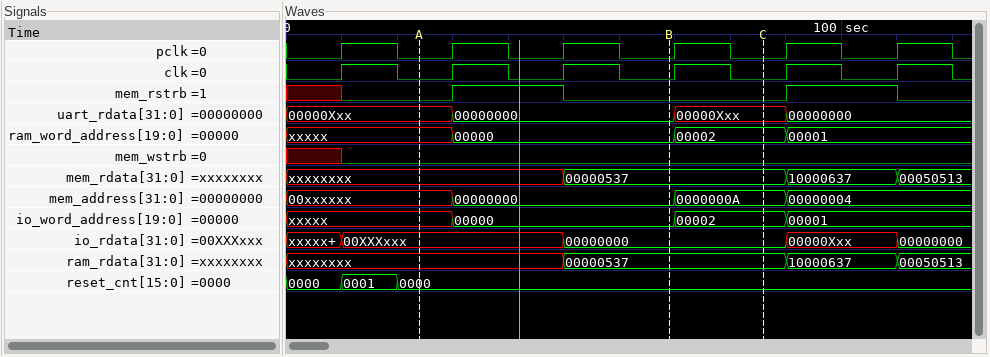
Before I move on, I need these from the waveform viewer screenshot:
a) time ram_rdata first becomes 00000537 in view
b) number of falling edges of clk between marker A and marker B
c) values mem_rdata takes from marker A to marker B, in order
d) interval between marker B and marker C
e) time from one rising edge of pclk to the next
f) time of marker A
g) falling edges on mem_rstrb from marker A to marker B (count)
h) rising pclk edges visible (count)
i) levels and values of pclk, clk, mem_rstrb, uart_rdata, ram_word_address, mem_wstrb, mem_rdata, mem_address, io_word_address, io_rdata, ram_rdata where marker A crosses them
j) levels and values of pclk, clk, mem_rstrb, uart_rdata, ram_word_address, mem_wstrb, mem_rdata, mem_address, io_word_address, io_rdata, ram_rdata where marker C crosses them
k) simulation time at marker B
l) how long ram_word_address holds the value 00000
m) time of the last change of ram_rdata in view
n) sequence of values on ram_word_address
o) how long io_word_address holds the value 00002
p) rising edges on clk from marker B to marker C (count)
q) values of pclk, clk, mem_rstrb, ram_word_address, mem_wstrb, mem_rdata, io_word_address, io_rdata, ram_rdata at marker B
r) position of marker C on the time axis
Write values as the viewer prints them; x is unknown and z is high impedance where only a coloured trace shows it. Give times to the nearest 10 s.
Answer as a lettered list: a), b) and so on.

a) 50 s
b) 2
c) xxxxxxxx, 00000537
d) 20 s
e) 20 s
f) 20 s
g) 1
h) 6
i) pclk=0, clk=0, mem_rstrb=0, uart_rdata=00000Xxx, ram_word_address=xxxxx, mem_wstrb=0, mem_rdata=xxxxxxxx, mem_address=00xxxxxx, io_word_address=xxxxx, io_rdata=00XXXxxx, ram_rdata=xxxxxxxx
j) pclk=0, clk=0, mem_rstrb=0, uart_rdata=00000Xxx, ram_word_address=00002, mem_wstrb=0, mem_rdata=00000537, mem_address=0000000A, io_word_address=00002, io_rdata=00000000, ram_rdata=00000537
k) 70 s
l) 40 s
m) 110 s
n) xxxxx, 00000, 00002, 00001
o) 20 s
p) 1
q) pclk=0, clk=0, mem_rstrb=0, ram_word_address=00000, mem_wstrb=0, mem_rdata=00000537, io_word_address=00000, io_rdata=00000000, ram_rdata=00000537
r) 90 s
